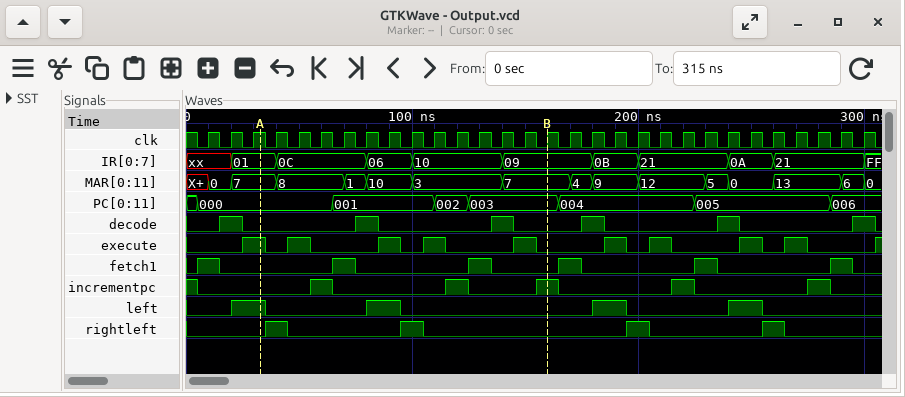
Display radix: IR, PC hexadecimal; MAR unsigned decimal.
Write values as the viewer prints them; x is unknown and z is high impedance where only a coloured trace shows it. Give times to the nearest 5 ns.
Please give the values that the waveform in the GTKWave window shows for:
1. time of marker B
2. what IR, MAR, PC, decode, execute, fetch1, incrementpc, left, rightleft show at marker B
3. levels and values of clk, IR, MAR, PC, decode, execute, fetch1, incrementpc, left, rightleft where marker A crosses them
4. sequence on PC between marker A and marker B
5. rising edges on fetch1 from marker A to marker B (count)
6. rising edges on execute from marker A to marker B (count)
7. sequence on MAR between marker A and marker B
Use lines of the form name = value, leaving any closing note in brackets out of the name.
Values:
time of marker B = 160 ns
what IR, MAR, PC, decode, execute, fetch1, incrementpc, left, rightleft show at marker B = IR=09, MAR=7, PC=003, decode=0, execute=0, fetch1=0, incrementpc=1, left=0, rightleft=0
levels and values of clk, IR, MAR, PC, decode, execute, fetch1, incrementpc, left, rightleft where marker A crosses them = clk=1, IR=01, MAR=7, PC=000, decode=0, execute=1, fetch1=0, incrementpc=0, left=1, rightleft=0
sequence on PC between marker A and marker B = 000, 001, 002, 003
rising edges on fetch1 from marker A to marker B = 2
rising edges on execute from marker A to marker B = 4
sequence on MAR between marker A and marker B = 7, 8, 1, 10, 3, 7
